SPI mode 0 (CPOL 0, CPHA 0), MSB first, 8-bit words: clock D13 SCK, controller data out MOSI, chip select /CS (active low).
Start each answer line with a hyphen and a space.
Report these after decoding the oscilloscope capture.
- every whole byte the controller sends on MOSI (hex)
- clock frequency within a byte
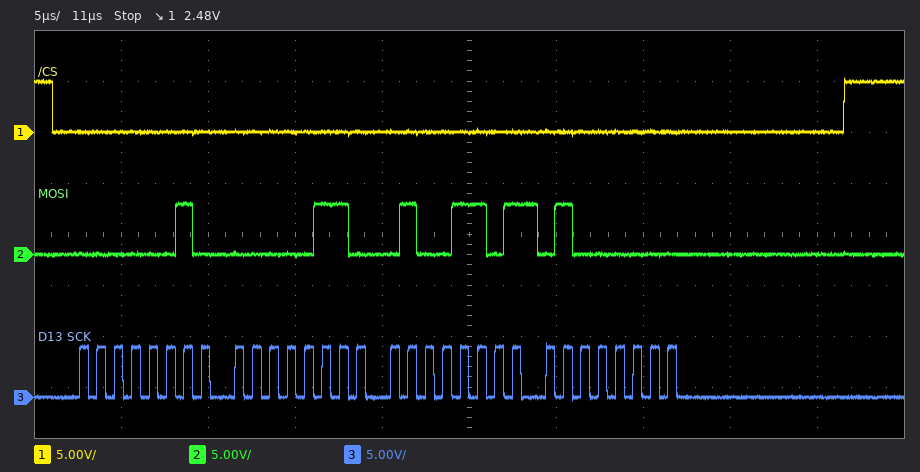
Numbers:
- 0x02 0x06 0x4D 0x40
- 1 MHz
